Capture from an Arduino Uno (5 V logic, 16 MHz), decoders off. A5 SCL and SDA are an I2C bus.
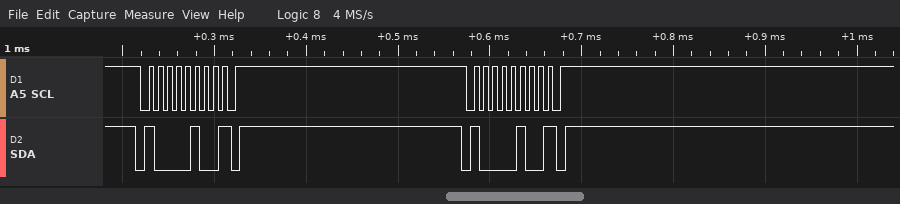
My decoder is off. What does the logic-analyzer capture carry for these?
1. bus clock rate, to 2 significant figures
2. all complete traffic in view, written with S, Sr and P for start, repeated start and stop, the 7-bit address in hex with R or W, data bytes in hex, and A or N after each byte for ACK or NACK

100 kHz
S 42W N P S 42W N P
